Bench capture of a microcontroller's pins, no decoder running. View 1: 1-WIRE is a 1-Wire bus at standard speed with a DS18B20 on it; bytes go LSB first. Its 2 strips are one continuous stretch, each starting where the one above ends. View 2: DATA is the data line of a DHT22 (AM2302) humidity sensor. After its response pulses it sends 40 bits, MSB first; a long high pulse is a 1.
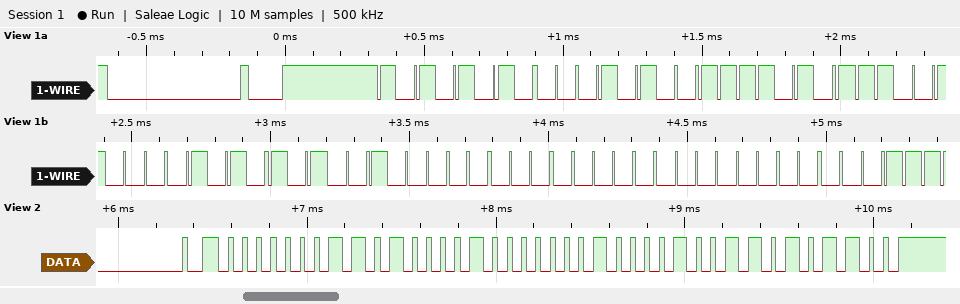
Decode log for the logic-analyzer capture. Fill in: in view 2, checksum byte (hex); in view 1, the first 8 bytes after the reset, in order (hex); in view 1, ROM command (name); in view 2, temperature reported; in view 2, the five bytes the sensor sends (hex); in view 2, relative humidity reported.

0xAC
55 28 AF 13 AA 04 00 00
Match ROM
26.5 °C
01 A1 01 09 AC
41.7 %
